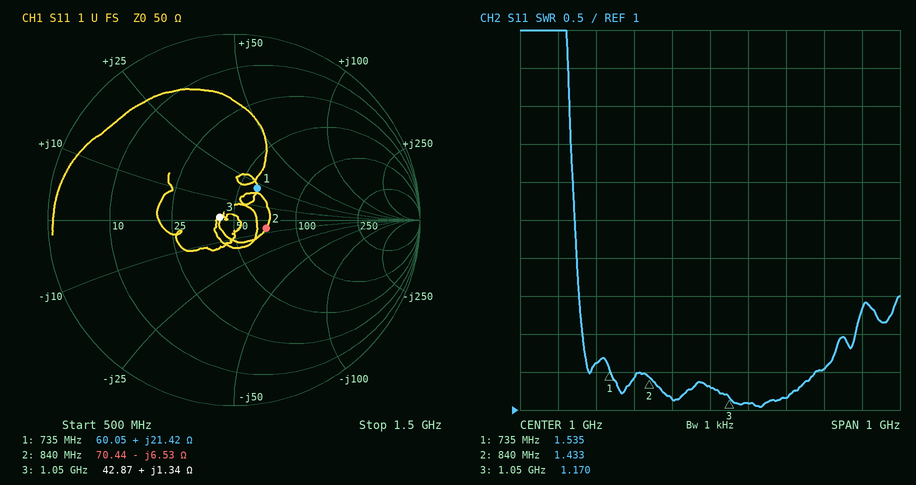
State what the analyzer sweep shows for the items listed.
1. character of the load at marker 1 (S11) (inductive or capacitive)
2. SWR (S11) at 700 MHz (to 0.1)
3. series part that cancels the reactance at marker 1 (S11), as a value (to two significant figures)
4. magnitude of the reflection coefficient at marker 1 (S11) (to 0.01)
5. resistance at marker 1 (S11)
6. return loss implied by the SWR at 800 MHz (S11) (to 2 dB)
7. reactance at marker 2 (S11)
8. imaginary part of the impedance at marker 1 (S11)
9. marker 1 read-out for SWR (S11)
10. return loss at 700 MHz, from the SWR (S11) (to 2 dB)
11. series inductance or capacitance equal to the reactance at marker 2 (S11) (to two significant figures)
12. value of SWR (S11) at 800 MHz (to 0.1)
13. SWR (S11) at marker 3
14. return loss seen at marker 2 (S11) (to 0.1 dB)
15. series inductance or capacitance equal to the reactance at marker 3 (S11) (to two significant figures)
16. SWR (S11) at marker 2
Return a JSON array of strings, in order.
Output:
["inductive", "1.6", "10 pF", "0.21", "60.05 Ω", "16 dB", "-6.53 Ω", "+21.42 Ω", "1.535", "12 dB", "29 pF", "1.4", "1.170", "15.0 dB", "200 pH", "1.433"]
